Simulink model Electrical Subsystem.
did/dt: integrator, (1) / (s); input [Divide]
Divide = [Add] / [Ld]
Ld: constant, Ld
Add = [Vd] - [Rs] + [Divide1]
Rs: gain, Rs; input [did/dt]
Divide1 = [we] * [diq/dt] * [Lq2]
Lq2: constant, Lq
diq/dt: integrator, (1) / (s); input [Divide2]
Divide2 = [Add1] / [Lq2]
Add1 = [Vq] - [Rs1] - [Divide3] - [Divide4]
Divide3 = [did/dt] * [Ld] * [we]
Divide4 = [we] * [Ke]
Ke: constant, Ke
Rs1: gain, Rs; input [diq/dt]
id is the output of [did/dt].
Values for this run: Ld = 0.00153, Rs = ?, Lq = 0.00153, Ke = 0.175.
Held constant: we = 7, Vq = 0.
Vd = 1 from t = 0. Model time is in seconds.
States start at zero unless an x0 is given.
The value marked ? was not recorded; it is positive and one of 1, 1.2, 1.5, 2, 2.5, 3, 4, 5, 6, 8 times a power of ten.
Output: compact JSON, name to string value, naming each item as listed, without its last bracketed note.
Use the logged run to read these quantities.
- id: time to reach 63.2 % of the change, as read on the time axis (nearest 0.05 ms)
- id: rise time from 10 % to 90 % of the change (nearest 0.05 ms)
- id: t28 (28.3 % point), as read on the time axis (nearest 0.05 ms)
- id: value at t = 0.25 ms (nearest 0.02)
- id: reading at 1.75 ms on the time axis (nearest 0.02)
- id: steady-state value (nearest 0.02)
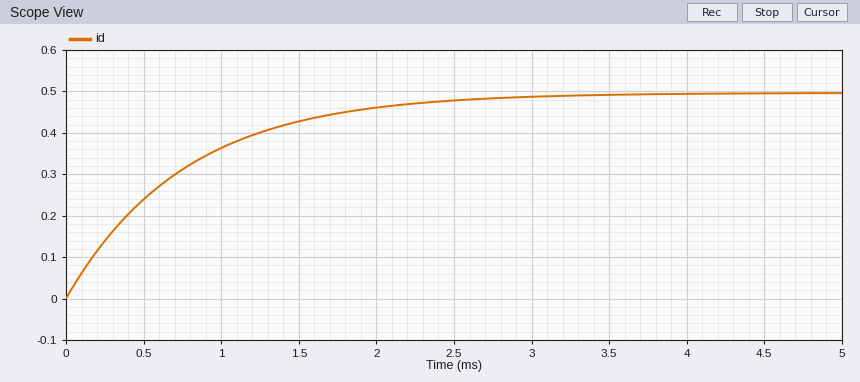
{"id: time to reach 63.2 % of the change, as read on the time axis": "0.75 ms", "id: rise time from 10 % to 90 % of the change": "1.65 ms", "id: t28 (28.3 % point), as read on the time axis": "0.25 ms", "id: value at t = 0.25 ms": "0.14", "id: reading at 1.75 ms on the time axis": "0.44", "id: steady-state value": "0.50"}
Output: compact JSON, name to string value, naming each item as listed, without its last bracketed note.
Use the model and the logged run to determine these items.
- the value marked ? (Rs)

{"the value marked ?": "2"}
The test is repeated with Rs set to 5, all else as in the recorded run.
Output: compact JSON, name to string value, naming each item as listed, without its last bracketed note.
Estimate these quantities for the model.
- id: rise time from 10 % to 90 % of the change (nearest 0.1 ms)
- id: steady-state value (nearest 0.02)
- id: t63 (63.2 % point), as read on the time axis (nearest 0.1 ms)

{"id: rise time from 10 % to 90 % of the change": "0.7 ms", "id: steady-state value": "0.20", "id: t63 (63.2 % point), as read on the time axis": "0.3 ms"}
